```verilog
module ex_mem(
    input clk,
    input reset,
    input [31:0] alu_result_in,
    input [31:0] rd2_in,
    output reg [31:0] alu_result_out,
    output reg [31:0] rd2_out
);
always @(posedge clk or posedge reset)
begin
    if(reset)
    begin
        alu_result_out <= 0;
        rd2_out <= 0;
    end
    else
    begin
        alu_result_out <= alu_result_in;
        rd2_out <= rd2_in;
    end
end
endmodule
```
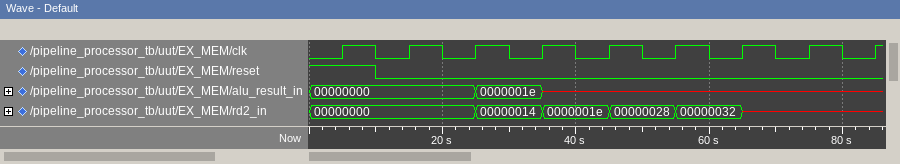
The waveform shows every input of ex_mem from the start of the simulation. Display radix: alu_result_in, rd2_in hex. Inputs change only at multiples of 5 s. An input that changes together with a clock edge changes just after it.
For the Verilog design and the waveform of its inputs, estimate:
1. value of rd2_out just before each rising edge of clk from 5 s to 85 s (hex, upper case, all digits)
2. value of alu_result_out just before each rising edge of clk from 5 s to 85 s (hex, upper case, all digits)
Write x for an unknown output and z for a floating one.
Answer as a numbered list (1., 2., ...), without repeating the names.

1. 00000000, 00000000, 00000000, 00000000, 00000014, 0000001E, 00000028, 00000032, x
2. 00000000, 00000000, 00000000, 00000000, 0000001E, x, x, x, x
